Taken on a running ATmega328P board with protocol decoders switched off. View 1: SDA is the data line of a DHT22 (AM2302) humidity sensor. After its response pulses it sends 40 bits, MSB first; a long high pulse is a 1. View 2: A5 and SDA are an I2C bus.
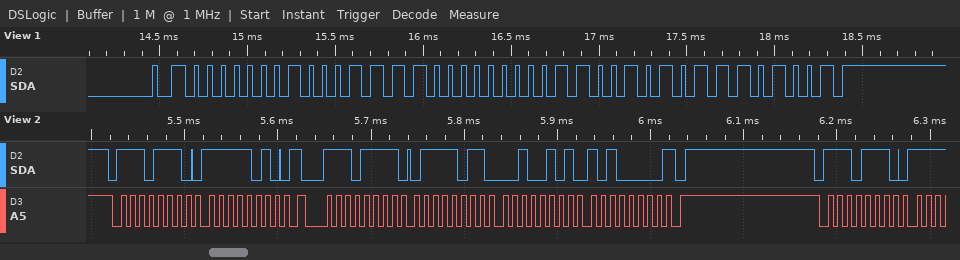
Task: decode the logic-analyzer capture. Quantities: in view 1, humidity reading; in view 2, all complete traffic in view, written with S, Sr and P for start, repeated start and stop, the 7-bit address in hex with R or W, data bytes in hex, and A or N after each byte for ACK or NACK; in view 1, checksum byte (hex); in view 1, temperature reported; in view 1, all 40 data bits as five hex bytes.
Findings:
28.6 %
S 77W A FA A Sr 77R A 7B A 25 A A0 N P S 77W A
0xE9
20.2 °C
01 1E 00 CA E9
